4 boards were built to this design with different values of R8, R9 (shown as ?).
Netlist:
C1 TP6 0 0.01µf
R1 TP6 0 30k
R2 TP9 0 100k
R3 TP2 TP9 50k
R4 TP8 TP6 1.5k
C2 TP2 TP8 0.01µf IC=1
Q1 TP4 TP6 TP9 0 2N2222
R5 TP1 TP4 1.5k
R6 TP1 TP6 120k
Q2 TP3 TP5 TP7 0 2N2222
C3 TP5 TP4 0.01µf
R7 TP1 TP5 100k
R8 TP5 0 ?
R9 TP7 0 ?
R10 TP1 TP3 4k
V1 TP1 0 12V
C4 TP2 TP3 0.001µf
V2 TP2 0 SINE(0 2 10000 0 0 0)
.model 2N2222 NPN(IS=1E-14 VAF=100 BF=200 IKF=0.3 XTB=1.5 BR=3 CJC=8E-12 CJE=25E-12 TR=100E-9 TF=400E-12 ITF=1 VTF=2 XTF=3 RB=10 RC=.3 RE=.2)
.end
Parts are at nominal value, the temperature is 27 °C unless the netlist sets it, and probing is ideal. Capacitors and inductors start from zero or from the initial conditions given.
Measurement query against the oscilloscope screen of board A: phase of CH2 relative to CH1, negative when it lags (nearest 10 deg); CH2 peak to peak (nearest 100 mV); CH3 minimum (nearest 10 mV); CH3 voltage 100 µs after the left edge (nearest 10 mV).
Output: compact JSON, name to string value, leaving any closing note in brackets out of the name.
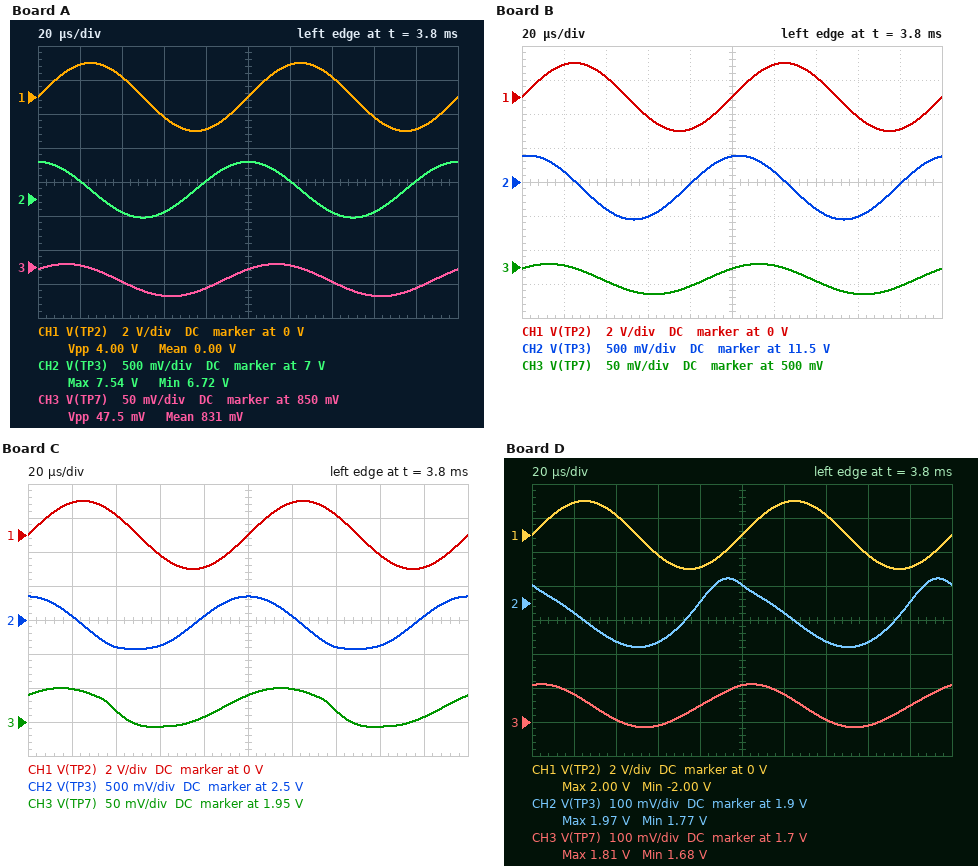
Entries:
{"phase of CH2 relative to CH1, negative when it lags": "90 deg", "CH2 peak to peak": "800 mV", "CH3 minimum": "810 mV", "CH3 voltage 100 µs after the left edge": "850 mV"}
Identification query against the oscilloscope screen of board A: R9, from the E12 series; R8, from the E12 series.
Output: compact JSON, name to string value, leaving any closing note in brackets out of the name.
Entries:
{"R9, from the E12 series": "680 Ω", "R8, from the E12 series": "15 kΩ"}
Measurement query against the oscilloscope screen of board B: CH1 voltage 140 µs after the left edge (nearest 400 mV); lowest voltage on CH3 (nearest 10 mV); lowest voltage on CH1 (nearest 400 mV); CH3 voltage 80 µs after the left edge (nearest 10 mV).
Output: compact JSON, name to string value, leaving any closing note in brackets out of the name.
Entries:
{"CH1 voltage 140 µs after the left edge": "1.2 V", "lowest voltage on CH3": "460 mV", "lowest voltage on CH1": "-2.0 V", "CH3 voltage 80 µs after the left edge": "470 mV"}
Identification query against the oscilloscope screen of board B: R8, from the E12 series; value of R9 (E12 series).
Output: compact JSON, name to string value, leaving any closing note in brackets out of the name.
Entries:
{"R8, from the E12 series": "10 kΩ", "value of R9": "3.3 kΩ"}
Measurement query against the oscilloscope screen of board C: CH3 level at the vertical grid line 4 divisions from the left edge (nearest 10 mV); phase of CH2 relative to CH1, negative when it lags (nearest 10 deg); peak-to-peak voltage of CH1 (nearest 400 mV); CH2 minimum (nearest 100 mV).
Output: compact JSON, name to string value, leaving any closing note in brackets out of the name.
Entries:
{"CH3 level at the vertical grid line 4 divisions from the left edge": "1.96 V", "phase of CH2 relative to CH1, negative when it lags": "90 deg", "peak-to-peak voltage of CH1": "4.0 V", "CH2 minimum": "2.1 V"}
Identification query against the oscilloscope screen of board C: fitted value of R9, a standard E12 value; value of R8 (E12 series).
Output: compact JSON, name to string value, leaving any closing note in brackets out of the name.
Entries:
{"fitted value of R9, a standard E12 value": "820 Ω", "value of R8": "33 kΩ"}
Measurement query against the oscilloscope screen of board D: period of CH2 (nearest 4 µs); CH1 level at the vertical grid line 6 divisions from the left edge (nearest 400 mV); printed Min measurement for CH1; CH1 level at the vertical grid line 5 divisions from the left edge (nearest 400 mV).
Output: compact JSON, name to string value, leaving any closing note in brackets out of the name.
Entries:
{"period of CH2": "100 µs", "CH1 level at the vertical grid line 6 divisions from the left edge": "2.0 V", "printed Min measurement for CH1": "-2.00 V", "CH1 level at the vertical grid line 5 divisions from the left edge": "0 V"}
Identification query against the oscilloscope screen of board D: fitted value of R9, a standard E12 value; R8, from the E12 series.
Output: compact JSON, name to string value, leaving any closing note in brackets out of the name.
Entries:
{"fitted value of R9, a standard E12 value": "680 Ω", "R8, from the E12 series": "39 kΩ"}
